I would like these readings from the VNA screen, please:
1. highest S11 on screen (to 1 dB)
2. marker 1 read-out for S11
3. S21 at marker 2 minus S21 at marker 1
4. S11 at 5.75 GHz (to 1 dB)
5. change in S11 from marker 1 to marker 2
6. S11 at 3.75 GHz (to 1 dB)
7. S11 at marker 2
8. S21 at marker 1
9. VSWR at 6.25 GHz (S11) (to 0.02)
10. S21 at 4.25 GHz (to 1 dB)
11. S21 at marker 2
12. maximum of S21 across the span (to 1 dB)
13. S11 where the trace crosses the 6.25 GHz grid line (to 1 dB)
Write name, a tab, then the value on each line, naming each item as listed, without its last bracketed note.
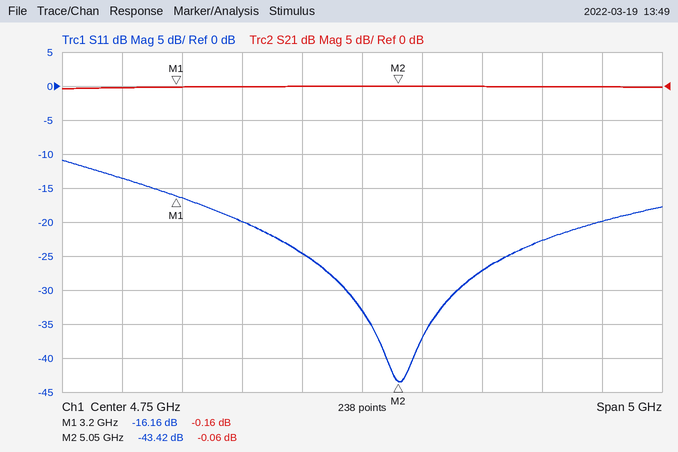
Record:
highest S11 on screen	-11 dB
marker 1 read-out for S11	-16.16 dB
S21 at marker 2 minus S21 at marker 1	0.10 dB
S11 at 5.75 GHz	-27 dB
change in S11 from marker 1 to marker 2	-27.26 dB
S11 at 3.75 GHz	-20 dB
S11 at marker 2	-43.42 dB
S21 at marker 1	-0.16 dB
VSWR at 6.25 GHz (S11)	1.16
S21 at 4.25 GHz	0 dB
S21 at marker 2	-0.06 dB
maximum of S21 across the span	0 dB
S11 where the trace crosses the 6.25 GHz grid line	-23 dB
